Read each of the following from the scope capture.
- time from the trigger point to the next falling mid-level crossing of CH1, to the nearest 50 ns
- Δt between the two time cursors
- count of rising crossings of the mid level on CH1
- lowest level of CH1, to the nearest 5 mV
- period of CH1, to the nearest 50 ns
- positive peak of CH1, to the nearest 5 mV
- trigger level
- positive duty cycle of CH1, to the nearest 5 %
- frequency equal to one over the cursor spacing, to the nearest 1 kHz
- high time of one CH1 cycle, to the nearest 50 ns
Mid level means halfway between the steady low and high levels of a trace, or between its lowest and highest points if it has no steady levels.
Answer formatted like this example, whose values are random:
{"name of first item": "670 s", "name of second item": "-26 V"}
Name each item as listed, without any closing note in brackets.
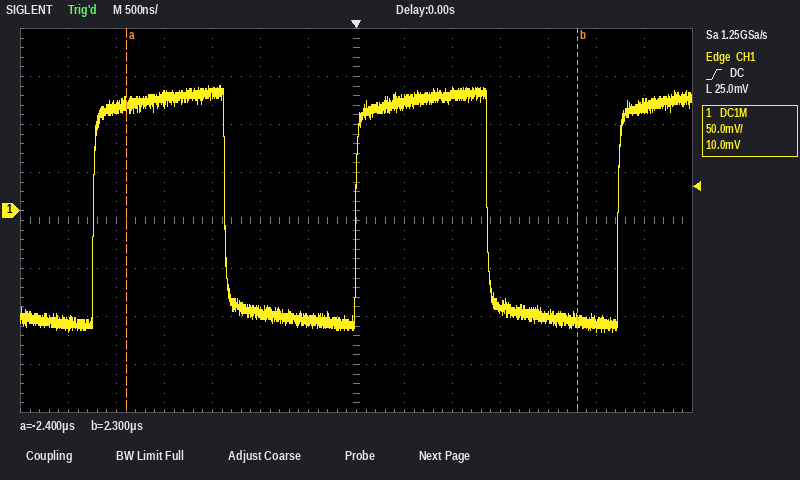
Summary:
{"time from the trigger point to the next falling mid-level crossing of CH1, to the nearest 50 ns": "1.35 µs", "Δt between the two time cursors": "4.70 µs", "count of rising crossings of the mid level on CH1": "3", "lowest level of CH1, to the nearest 5 mV": "-125 mV", "period of CH1, to the nearest 50 ns": "2.75 µs", "positive peak of CH1, to the nearest 5 mV": "130 mV", "trigger level": "25.0 mV", "positive duty cycle of CH1, to the nearest 5 %": "50 %", "frequency equal to one over the cursor spacing, to the nearest 1 kHz": "213 kHz", "high time of one CH1 cycle, to the nearest 50 ns": "1.35 µs"}
